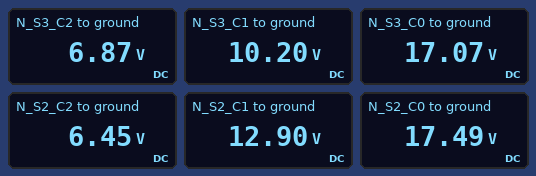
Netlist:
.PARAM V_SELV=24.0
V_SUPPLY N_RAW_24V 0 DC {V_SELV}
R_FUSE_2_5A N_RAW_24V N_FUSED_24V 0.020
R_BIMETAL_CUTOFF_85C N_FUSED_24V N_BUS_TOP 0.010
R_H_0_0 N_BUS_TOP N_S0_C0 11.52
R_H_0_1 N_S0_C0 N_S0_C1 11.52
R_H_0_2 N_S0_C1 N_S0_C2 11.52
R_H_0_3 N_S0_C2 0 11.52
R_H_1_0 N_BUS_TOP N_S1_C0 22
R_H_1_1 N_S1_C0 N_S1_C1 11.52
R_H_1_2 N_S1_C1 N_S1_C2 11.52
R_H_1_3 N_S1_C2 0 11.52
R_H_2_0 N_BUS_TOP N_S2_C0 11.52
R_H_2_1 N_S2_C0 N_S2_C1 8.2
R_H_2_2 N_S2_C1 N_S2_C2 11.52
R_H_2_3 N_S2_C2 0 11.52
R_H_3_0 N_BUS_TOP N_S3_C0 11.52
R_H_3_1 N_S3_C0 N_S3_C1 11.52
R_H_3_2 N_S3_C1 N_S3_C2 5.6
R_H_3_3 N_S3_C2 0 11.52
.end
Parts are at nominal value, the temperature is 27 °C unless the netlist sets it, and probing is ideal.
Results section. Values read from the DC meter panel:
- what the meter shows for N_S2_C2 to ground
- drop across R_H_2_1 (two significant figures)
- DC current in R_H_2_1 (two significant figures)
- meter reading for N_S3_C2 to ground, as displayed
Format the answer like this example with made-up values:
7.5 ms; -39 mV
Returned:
6.45 V; 4.6 V; 560 mA; 6.87 V
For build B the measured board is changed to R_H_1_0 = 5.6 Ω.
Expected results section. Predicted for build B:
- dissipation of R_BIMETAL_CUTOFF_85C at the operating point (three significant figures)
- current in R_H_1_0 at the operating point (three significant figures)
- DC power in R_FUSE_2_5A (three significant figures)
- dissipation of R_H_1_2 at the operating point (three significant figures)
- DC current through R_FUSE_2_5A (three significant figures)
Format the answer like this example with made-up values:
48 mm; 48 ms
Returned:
51.6 mW; 596 mA; 103 mW; 4.09 W; 2.27 A
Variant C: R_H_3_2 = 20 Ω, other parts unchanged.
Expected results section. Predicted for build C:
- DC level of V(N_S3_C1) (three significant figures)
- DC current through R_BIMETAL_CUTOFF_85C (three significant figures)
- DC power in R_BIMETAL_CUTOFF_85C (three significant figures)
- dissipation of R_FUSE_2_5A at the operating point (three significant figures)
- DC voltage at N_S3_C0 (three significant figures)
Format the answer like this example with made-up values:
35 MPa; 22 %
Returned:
13.8 V; 1.94 A; 37.7 mW; 75.4 mW; 18.9 V
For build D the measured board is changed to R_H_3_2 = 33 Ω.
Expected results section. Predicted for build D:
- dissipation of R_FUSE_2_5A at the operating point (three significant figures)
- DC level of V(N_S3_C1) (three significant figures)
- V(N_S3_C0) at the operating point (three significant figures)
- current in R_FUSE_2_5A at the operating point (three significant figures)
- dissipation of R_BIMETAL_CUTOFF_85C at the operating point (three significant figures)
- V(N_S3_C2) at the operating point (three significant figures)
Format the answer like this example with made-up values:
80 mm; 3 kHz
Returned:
69.0 mW; 15.8 V; 19.9 V; 1.86 A; 34.5 mW; 4.08 V
